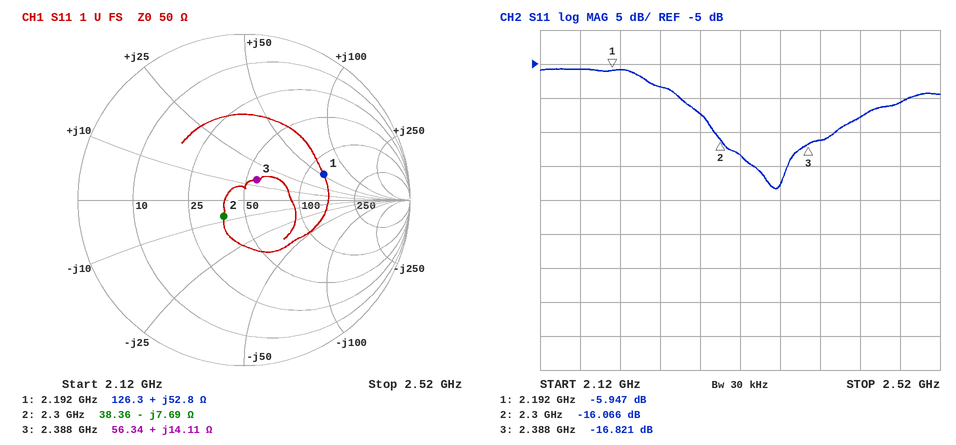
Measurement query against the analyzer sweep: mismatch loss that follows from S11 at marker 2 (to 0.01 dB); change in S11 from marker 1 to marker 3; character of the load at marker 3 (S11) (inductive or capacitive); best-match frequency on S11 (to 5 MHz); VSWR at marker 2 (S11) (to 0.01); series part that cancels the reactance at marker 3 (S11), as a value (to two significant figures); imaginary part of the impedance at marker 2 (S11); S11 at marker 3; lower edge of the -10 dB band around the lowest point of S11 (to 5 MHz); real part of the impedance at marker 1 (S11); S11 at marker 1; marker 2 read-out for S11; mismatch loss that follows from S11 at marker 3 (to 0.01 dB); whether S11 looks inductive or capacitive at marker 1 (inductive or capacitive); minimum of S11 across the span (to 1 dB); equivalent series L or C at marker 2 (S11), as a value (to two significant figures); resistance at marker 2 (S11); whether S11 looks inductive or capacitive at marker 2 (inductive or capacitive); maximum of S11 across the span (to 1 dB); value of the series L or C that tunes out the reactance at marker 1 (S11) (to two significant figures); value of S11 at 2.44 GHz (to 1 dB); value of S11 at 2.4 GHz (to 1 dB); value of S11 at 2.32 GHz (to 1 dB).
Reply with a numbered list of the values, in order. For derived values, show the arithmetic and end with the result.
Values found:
1. −10 log10(1 − 10^(-16.066/10)) ≈ 0.11 dB
2. -16.821 − (-5.947) = -10.874 dB
3. inductive
4. 2.355 GHz
5. 1.37
6. C = 1/(2π × 2.388 GHz × 14.11 Ω) ≈ 4.7 pF
7. -7.69 Ω
8. -16.821 dB
9. 2.260 GHz
10. 126.3 Ω
11. -5.947 dB
12. -16.066 dB
13. −10 log10(1 − 10^(-16.821/10)) ≈ 0.09 dB
14. inductive
15. -23 dB
16. C = 1/(2π × 2.3 GHz × 7.69 Ω) ≈ 9.0 pF
17. 38.36 Ω
18. capacitive
19. -6 dB
20. C = 1/(2π × 2.192 GHz × 52.8 Ω) ≈ 1.4 pF
21. -13 dB
22. -16 dB
23. -18 dB
